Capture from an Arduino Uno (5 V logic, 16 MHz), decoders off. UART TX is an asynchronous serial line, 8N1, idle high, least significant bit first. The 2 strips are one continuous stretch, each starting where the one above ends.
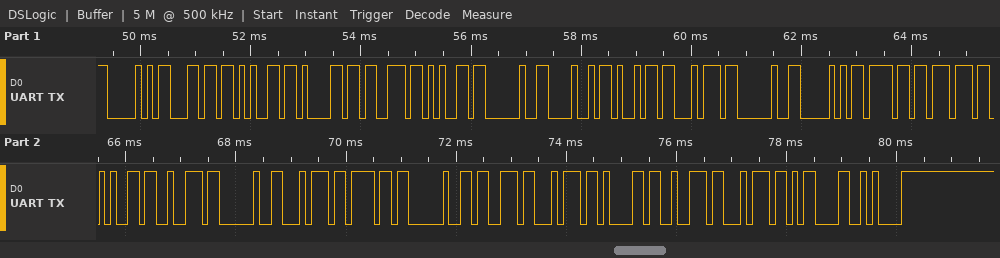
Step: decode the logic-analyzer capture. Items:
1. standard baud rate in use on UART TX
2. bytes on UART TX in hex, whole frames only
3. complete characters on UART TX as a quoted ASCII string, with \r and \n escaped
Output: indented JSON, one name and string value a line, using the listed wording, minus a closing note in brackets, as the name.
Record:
{
  "standard baud rate in use on UART TX": "9600 baud",
  "bytes on UART TX in hex, whole frames only": "50 6C 65 61 73 65 20 48 69 74 20 50 6F 77 65 72 20 74 6F 20 73 74 61 72 74 0D 0A",
  "complete characters on UART TX as a quoted ASCII string, with \\r and \\n escaped": "\"Please Hit Power to start\\r\\n\""
}
